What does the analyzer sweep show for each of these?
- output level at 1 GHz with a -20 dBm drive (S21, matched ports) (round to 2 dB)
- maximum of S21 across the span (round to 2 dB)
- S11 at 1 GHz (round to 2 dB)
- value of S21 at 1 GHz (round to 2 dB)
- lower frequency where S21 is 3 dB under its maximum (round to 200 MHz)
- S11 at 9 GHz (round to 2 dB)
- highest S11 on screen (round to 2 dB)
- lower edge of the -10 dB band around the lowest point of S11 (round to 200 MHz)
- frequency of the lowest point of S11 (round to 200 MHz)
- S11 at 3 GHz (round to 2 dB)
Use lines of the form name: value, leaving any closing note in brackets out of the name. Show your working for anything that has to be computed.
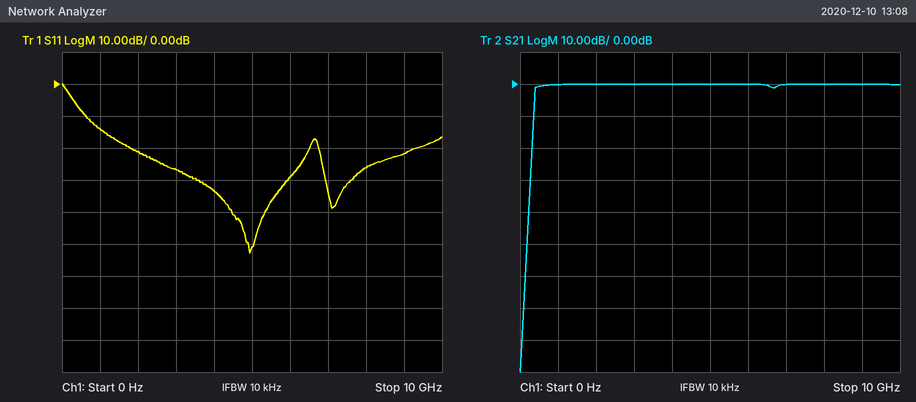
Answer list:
output level at 1 GHz with a -20 dBm drive (S21, matched ports): -20 dBm + (0 dB) = -20 dBm
maximum of S21 across the span: 0 dB
S11 at 1 GHz: -14 dB
value of S21 at 1 GHz: 0 dB
lower frequency where S21 is 3 dB under its maximum: 400 MHz
S11 at 9 GHz: -22 dB
highest S11 on screen: 0 dB
lower edge of the -10 dB band around the lowest point of S11: 600 MHz
frequency of the lowest point of S11: 5.0 GHz
S11 at 3 GHz: -26 dB
